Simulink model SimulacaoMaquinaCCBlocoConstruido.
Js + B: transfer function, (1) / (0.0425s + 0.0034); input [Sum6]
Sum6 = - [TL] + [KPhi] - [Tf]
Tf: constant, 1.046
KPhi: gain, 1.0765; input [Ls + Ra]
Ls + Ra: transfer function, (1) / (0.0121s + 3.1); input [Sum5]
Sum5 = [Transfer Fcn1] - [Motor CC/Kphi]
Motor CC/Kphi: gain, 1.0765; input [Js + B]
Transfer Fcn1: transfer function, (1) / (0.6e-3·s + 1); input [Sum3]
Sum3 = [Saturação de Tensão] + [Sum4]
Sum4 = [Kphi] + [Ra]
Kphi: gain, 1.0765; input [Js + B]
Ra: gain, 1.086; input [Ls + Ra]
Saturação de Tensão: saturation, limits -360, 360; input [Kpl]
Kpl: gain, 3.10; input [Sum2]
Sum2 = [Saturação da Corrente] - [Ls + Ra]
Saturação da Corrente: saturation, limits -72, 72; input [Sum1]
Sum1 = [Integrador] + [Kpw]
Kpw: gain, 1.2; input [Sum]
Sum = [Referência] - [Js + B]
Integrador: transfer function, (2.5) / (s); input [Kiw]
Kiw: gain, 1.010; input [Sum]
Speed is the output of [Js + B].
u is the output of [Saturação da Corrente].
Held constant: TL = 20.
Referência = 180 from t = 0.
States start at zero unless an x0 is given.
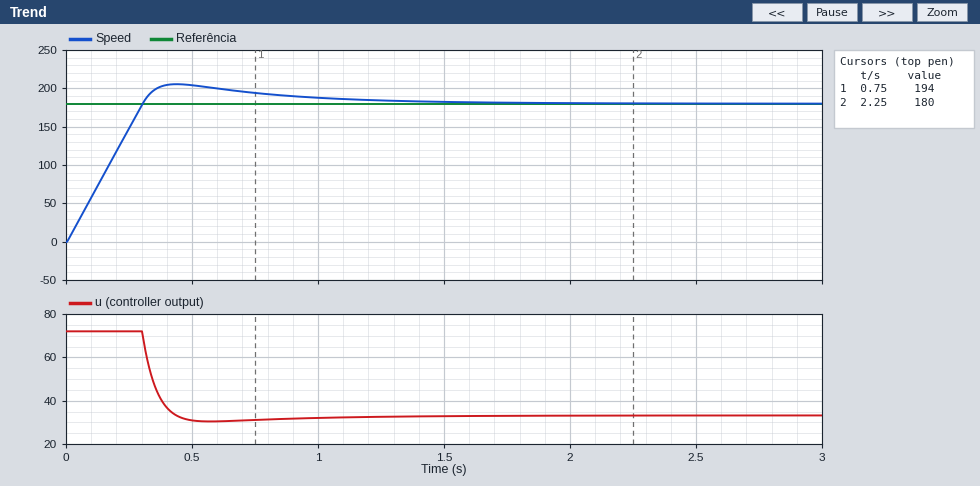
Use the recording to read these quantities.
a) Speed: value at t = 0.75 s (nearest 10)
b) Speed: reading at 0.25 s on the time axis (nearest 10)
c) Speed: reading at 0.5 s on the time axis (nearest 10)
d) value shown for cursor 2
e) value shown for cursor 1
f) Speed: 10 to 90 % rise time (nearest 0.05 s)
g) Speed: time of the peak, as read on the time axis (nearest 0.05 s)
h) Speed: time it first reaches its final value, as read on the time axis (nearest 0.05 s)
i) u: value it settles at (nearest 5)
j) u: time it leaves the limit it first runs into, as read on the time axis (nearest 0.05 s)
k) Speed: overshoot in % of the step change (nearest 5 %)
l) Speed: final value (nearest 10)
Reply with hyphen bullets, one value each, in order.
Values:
- 190
- 150
- 200
- 180
- 194
- 0.25 s
- 0.45 s
- 0.30 s
- 35
- 0.30 s
- 15 %
- 180
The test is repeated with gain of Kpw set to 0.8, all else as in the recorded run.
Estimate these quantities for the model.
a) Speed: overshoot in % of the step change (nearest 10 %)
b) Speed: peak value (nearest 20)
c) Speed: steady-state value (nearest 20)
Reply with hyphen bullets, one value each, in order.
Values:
- 20 %
- 220
- 180
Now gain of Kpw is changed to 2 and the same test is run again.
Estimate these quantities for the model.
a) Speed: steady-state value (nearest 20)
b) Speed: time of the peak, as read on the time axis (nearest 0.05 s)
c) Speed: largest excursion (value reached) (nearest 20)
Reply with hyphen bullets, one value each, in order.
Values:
- 180
- 0.40 s
- 200
